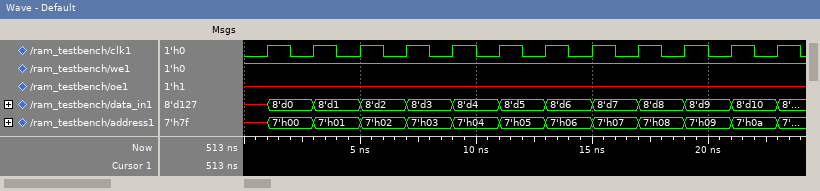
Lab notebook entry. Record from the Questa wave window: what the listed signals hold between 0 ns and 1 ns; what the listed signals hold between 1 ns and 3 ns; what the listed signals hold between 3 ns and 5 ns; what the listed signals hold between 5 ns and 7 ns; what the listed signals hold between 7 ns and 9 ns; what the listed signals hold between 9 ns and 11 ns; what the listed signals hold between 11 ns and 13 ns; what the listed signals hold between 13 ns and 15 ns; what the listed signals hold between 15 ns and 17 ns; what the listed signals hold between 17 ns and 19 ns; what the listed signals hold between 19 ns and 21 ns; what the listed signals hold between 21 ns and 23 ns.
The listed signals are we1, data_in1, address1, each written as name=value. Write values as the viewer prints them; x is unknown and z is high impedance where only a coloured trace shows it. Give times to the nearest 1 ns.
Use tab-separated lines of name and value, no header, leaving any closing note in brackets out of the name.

what the listed signals hold between 0 ns and 1 ns	we1=1, data_in1=x, address1=x
what the listed signals hold between 1 ns and 3 ns	we1=1, data_in1=8'd0, address1=7'h00
what the listed signals hold between 3 ns and 5 ns	we1=1, data_in1=8'd1, address1=7'h01
what the listed signals hold between 5 ns and 7 ns	we1=1, data_in1=8'd2, address1=7'h02
what the listed signals hold between 7 ns and 9 ns	we1=1, data_in1=8'd3, address1=7'h03
what the listed signals hold between 9 ns and 11 ns	we1=1, data_in1=8'd4, address1=7'h04
what the listed signals hold between 11 ns and 13 ns	we1=1, data_in1=8'd5, address1=7'h05
what the listed signals hold between 13 ns and 15 ns	we1=1, data_in1=8'd6, address1=7'h06
what the listed signals hold between 15 ns and 17 ns	we1=1, data_in1=8'd7, address1=7'h07
what the listed signals hold between 17 ns and 19 ns	we1=1, data_in1=8'd8, address1=7'h08
what the listed signals hold between 19 ns and 21 ns	we1=1, data_in1=8'd9, address1=7'h09
what the listed signals hold between 21 ns and 23 ns	we1=1, data_in1=8'd10, address1=7'h0a
